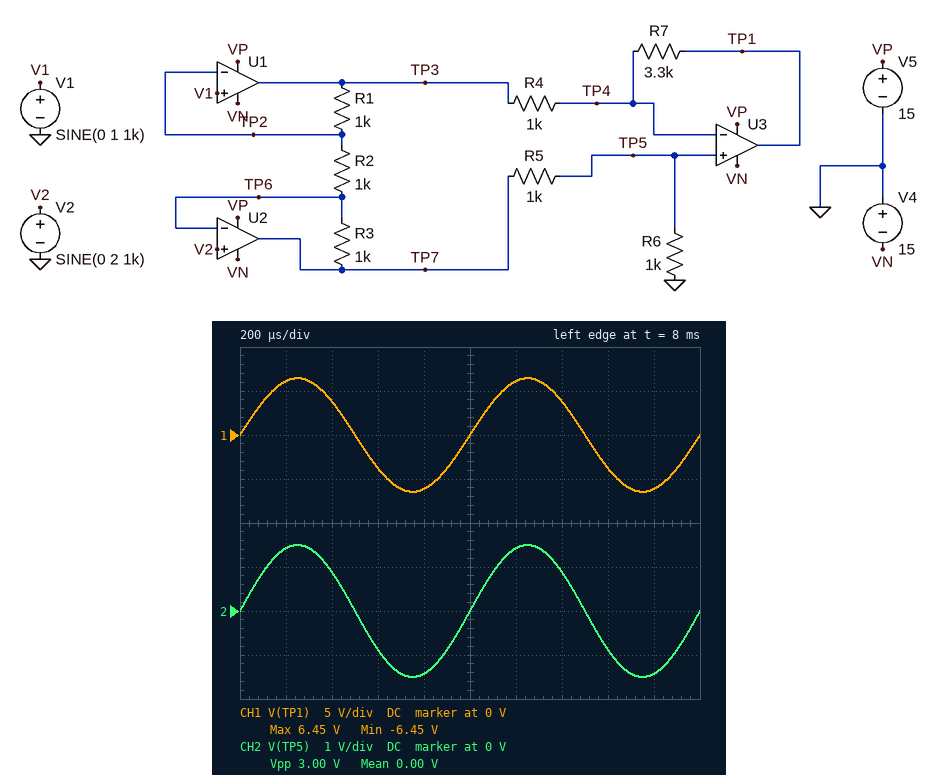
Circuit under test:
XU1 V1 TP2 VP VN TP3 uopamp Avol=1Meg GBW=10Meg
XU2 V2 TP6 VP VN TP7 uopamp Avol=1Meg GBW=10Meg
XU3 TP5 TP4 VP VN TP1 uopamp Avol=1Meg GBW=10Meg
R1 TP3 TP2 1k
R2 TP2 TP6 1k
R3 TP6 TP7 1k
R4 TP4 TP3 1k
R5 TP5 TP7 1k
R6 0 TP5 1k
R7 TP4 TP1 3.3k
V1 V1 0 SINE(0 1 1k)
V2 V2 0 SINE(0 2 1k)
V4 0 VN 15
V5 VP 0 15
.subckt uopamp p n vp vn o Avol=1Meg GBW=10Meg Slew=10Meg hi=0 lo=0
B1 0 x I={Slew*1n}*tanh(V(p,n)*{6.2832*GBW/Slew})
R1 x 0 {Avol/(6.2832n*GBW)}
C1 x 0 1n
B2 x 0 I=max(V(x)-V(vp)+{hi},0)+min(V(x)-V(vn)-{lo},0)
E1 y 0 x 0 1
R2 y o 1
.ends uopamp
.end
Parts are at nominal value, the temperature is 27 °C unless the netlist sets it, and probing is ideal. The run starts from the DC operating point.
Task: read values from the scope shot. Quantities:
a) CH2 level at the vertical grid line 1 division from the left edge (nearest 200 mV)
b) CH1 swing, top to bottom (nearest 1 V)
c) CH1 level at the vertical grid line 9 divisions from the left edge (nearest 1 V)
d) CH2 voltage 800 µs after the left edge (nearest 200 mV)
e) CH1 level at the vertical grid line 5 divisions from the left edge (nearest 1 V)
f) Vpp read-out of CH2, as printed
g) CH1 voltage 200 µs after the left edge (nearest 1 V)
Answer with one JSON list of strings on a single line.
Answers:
["1.4 V", "13 V", "-6 V", "-1.4 V", "0 V", "3.00 V", "6 V"]
